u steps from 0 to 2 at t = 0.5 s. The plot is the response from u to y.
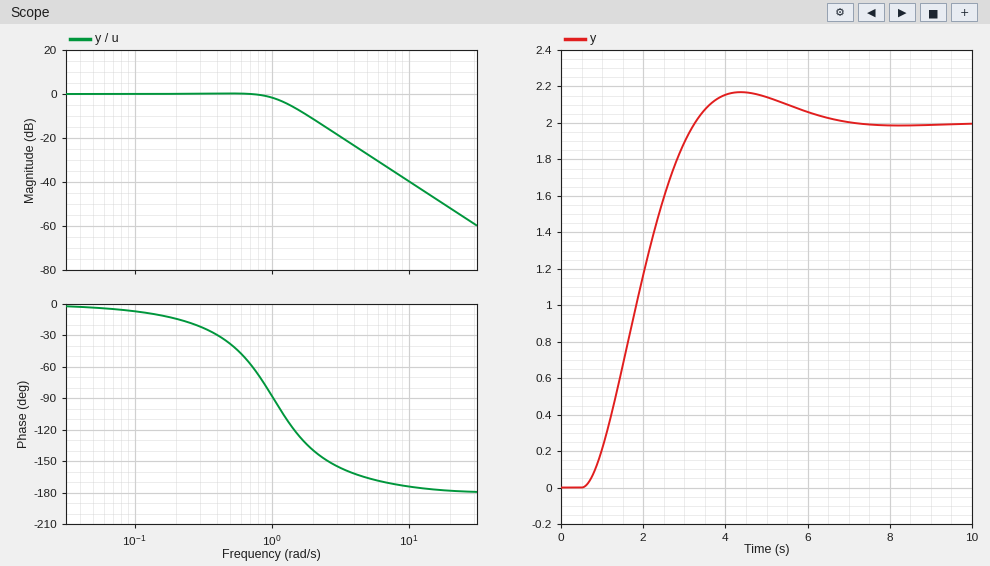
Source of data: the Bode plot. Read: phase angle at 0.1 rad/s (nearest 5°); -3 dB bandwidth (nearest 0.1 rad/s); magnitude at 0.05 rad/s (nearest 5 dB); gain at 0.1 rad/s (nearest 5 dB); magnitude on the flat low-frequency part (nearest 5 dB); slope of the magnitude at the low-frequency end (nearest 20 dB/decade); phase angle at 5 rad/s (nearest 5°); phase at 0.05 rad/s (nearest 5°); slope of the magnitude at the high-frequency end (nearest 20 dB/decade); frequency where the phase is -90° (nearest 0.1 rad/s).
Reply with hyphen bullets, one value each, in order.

- -5°
- 1.2 rad/s
- 0 dB
- 0 dB
- 0 dB
- 0 dB/decade
- -165°
- -5°
- -40 dB/decade
- 1.0 rad/s
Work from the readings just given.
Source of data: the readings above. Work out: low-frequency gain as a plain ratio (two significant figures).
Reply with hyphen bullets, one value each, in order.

- 1.0
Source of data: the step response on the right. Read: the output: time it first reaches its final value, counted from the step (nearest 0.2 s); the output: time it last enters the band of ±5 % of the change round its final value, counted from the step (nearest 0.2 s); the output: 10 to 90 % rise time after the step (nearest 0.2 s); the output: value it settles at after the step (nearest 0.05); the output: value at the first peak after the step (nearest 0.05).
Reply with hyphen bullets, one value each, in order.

- 2.8 s
- 5.0 s
- 1.8 s
- 2.00
- 2.15
